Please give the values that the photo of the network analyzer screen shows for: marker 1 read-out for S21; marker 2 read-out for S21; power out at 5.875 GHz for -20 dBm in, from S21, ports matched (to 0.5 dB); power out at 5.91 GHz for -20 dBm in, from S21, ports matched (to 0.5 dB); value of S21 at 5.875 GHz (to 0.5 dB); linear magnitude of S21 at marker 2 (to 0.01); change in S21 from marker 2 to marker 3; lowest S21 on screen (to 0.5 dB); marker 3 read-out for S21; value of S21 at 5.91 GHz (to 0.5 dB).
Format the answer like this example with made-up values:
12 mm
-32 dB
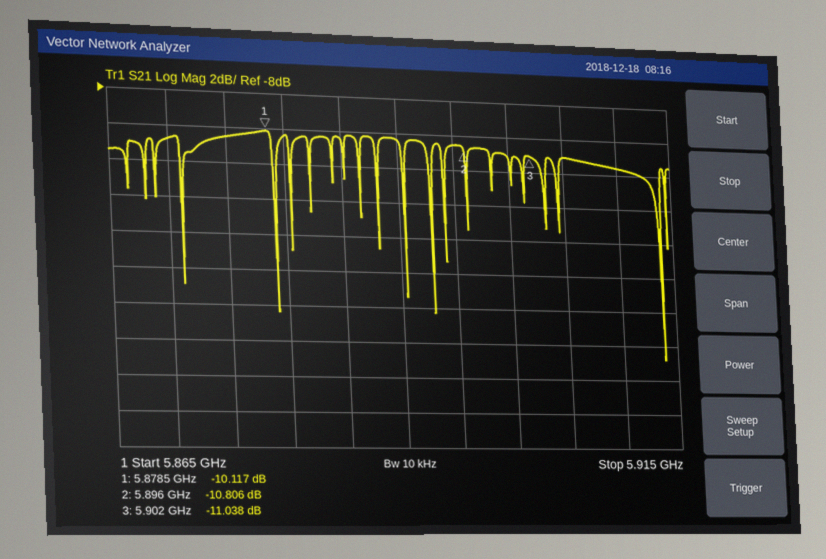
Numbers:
-10.117 dB
-10.806 dB
-30.5 dBm
-31.5 dBm
-10.5 dB
0.29
-0.232 dB
-23.0 dB
-11.038 dB
-11.5 dB
